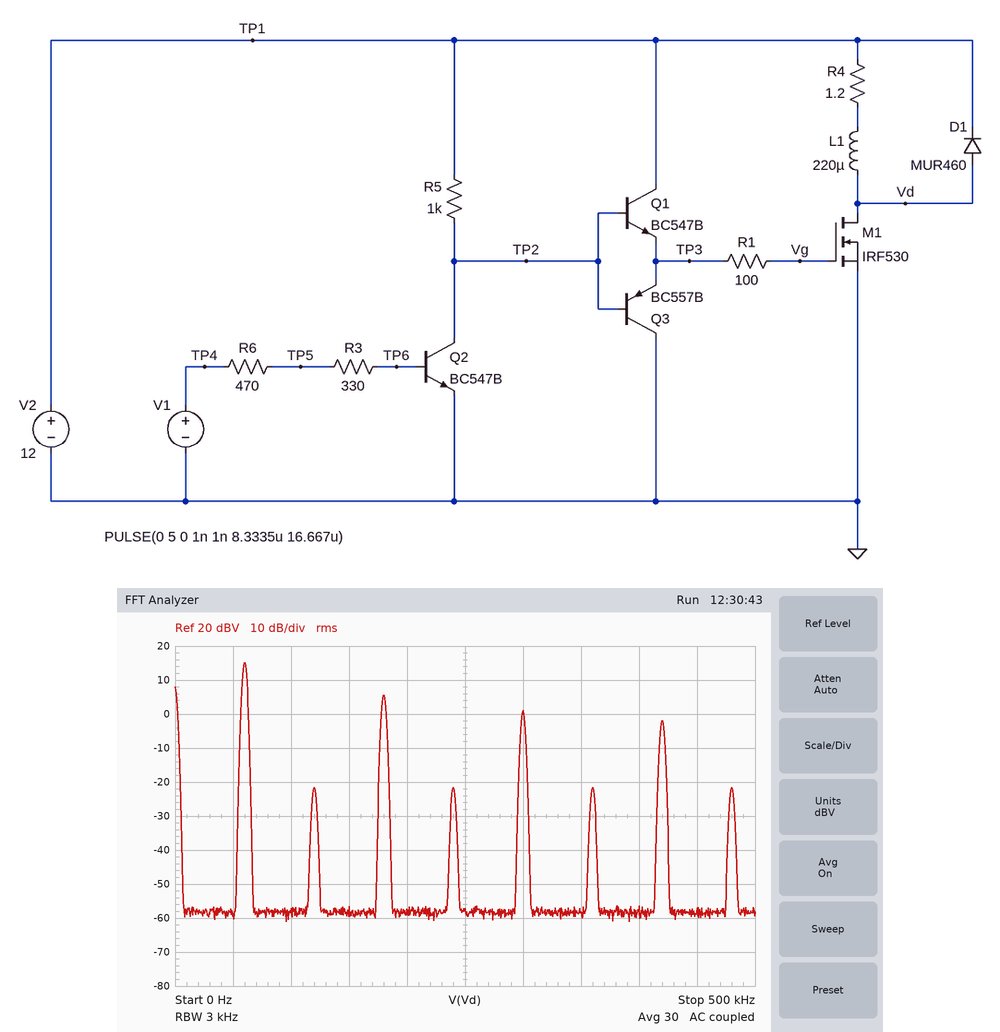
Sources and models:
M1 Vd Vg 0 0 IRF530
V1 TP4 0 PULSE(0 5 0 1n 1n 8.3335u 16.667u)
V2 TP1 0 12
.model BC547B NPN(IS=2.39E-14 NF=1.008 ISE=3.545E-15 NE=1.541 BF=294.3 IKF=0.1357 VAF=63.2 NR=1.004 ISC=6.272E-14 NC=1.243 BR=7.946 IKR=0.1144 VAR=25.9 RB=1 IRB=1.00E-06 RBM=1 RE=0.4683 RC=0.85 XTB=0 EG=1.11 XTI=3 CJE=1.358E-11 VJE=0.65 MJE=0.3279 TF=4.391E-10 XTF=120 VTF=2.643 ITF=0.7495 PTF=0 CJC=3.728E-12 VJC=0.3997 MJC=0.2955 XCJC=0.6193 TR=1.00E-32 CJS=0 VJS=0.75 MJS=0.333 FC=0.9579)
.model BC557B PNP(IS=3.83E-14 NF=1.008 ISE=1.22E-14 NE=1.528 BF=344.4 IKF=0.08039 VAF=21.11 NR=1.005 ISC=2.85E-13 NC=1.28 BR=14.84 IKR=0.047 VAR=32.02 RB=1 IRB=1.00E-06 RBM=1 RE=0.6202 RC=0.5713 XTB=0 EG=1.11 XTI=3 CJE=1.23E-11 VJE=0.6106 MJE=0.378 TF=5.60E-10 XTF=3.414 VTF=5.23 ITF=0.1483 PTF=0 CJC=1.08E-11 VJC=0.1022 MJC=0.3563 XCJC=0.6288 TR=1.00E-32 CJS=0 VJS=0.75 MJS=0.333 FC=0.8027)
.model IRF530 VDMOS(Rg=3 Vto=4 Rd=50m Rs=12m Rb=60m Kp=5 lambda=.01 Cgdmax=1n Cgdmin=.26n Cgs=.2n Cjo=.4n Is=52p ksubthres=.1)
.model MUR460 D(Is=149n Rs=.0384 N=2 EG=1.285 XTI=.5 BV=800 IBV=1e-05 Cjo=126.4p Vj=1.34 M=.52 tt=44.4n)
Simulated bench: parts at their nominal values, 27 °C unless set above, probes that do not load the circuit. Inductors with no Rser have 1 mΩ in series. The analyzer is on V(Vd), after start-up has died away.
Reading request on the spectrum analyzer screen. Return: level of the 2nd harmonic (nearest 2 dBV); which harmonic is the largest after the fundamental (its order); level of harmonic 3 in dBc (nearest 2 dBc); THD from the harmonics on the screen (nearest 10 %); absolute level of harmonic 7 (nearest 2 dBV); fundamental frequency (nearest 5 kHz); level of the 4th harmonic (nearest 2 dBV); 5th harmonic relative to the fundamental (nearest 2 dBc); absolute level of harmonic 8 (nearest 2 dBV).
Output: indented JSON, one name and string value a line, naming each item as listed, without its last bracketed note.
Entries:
{
  "level of the 2nd harmonic": "-22 dBV",
  "which harmonic is the largest after the fundamental": "3",
  "level of harmonic 3 in dBc": "-10 dBc",
  "THD from the harmonics on the screen": "40 %",
  "absolute level of harmonic 7": "-2 dBV",
  "fundamental frequency": "60 kHz",
  "level of the 4th harmonic": "-22 dBV",
  "5th harmonic relative to the fundamental": "-14 dBc",
  "absolute level of harmonic 8": "-22 dBV"
}
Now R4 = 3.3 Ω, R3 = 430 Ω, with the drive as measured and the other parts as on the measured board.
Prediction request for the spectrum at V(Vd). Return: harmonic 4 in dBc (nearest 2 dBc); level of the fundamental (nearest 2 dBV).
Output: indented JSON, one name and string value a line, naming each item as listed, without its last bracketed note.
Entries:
{
  "harmonic 4 in dBc": "-34 dBc",
  "level of the fundamental": "16 dBV"
}
